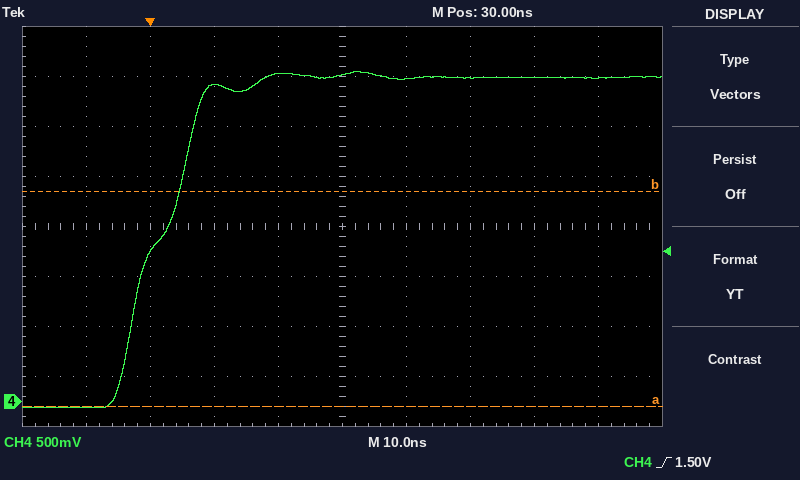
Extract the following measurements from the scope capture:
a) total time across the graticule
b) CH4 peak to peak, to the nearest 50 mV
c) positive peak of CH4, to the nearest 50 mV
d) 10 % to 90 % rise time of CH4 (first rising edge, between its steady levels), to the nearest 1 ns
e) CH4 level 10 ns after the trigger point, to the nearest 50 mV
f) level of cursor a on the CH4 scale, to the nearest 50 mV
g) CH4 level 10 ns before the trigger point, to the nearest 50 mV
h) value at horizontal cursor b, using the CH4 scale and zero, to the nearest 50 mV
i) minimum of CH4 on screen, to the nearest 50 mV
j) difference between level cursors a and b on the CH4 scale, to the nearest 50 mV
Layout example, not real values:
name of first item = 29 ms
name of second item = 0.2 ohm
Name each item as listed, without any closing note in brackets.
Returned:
total time across the graticule = 100 ns
CH4 peak to peak, to the nearest 50 mV = 3.35 V
positive peak of CH4, to the nearest 50 mV = 3.30 V
10 % to 90 % rise time of CH4 (first rising edge, between its steady levels), to the nearest 1 ns = 12 ns
CH4 level 10 ns after the trigger point, to the nearest 50 mV = 3.15 V
level of cursor a on the CH4 scale, to the nearest 50 mV = -50 mV
CH4 level 10 ns before the trigger point, to the nearest 50 mV = -50 mV
value at horizontal cursor b, using the CH4 scale and zero, to the nearest 50 mV = 2.10 V
minimum of CH4 on screen, to the nearest 50 mV = -50 mV
difference between level cursors a and b on the CH4 scale, to the nearest 50 mV = 2.15 V
